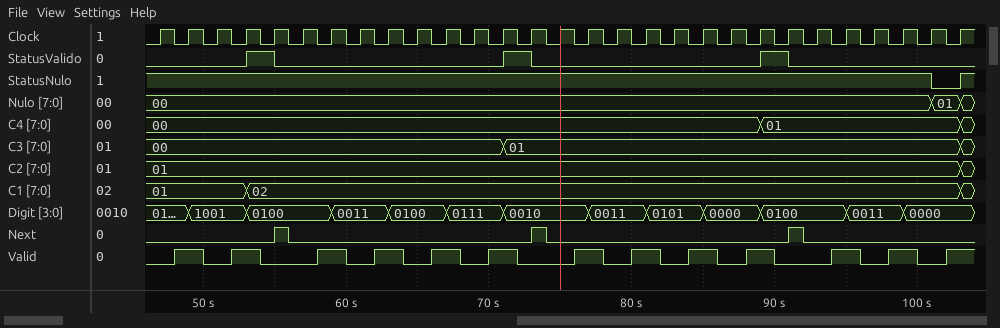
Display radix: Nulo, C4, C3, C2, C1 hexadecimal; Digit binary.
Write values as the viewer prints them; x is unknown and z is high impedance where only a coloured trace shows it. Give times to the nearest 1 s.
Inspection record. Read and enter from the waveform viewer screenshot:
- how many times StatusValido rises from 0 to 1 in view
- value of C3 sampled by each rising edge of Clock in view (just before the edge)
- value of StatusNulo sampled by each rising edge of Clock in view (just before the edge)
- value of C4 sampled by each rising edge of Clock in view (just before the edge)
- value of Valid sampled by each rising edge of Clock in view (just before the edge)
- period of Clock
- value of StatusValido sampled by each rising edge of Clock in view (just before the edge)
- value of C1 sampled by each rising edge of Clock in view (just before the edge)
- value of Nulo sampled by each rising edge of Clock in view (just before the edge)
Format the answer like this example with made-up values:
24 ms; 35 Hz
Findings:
3; 00, 00, 00, 00, 00, 00, 00, 00, 00, 00, 00, 00, 00, 01, 01, 01, 01, 01, 01, 01, 01, 01, 01, 01, 01, 01, 01, 01, 01; 1 1 1 1 1 1 1 1 1 1 1 1 1 1 1 1 1 1 1 1 1 1 1 1 1 1 1 1 0; 00, 00, 00, 00, 00, 00, 00, 00, 00, 00, 00, 00, 00, 00, 00, 00, 00, 00, 00, 00, 00, 00, 01, 01, 01, 01, 01, 01, 01; 0 1 0 1 0 0 1 0 1 0 1 0 1 0 0 1 0 1 0 1 0 1 0 0 1 0 1 0 1; 2 s; 0 0 0 0 1 0 0 0 0 0 0 0 0 1 0 0 0 0 0 0 0 0 1 0 0 0 0 0 0; 01, 01, 01, 01, 02, 02, 02, 02, 02, 02, 02, 02, 02, 02, 02, 02, 02, 02, 02, 02, 02, 02, 02, 02, 02, 02, 02, 02, 02; 00, 00, 00, 00, 00, 00, 00, 00, 00, 00, 00, 00, 00, 00, 00, 00, 00, 00, 00, 00, 00, 00, 00, 00, 00, 00, 00, 00, 01
